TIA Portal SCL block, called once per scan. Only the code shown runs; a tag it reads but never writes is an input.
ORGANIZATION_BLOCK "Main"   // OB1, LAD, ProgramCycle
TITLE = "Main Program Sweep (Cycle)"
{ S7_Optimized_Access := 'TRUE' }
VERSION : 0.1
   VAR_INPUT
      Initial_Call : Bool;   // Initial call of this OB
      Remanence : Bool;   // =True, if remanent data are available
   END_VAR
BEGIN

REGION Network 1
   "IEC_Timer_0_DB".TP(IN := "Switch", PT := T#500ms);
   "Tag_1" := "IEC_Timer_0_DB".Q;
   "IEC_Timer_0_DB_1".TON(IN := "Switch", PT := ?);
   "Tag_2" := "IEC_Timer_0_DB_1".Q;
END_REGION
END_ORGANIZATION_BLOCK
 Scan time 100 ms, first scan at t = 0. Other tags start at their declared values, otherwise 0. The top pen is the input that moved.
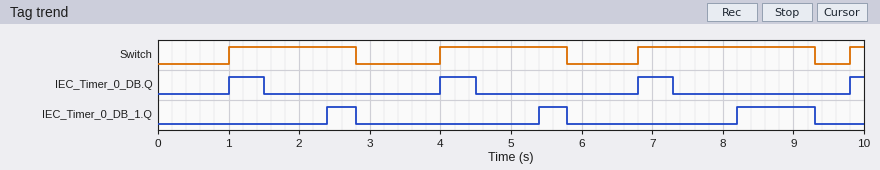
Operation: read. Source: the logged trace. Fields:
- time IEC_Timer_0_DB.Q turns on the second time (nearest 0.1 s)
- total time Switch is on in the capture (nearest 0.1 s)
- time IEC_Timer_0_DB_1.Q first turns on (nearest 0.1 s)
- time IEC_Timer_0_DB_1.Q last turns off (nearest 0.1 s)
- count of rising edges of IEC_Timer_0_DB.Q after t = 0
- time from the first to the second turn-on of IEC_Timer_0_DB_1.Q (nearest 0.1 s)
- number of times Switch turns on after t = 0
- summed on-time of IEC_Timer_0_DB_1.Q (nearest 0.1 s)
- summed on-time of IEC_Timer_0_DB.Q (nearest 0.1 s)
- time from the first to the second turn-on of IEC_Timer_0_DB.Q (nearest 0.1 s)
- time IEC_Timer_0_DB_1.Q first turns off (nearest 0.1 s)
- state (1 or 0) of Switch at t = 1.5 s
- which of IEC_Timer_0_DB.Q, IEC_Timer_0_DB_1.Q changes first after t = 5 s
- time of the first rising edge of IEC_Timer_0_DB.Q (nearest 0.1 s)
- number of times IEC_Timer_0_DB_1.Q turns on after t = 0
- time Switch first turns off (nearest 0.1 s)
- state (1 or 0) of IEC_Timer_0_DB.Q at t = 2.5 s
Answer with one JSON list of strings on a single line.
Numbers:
["4.0 s", "6.3 s", "2.4 s", "9.3 s", "4", "3.0 s", "4", "1.9 s", "1.7 s", "3.0 s", "2.8 s", "1", "IEC_Timer_0_DB_1.Q", "1.0 s", "3", "2.8 s", "0"]
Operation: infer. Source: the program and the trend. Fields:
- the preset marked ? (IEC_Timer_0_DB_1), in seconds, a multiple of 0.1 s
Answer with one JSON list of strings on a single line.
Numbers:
["1.4 s"]
